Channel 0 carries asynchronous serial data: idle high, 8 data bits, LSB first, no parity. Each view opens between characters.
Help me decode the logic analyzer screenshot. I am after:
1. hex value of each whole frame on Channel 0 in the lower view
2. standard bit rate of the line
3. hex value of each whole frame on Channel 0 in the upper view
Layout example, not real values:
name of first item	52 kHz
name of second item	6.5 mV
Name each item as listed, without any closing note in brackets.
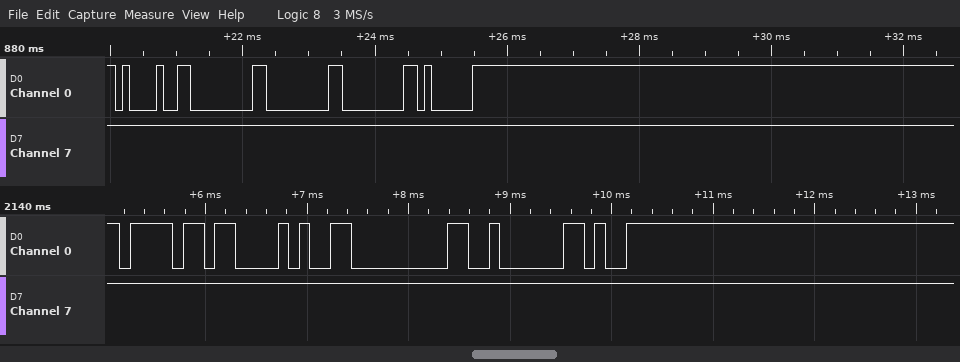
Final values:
hex value of each whole frame on Channel 0 in the lower view	6F, 28, 00, 02, F9
standard bit rate of the line	9600 baud
hex value of each whole frame on Channel 0 in the upper view	21, 00, 00, 00, 81
